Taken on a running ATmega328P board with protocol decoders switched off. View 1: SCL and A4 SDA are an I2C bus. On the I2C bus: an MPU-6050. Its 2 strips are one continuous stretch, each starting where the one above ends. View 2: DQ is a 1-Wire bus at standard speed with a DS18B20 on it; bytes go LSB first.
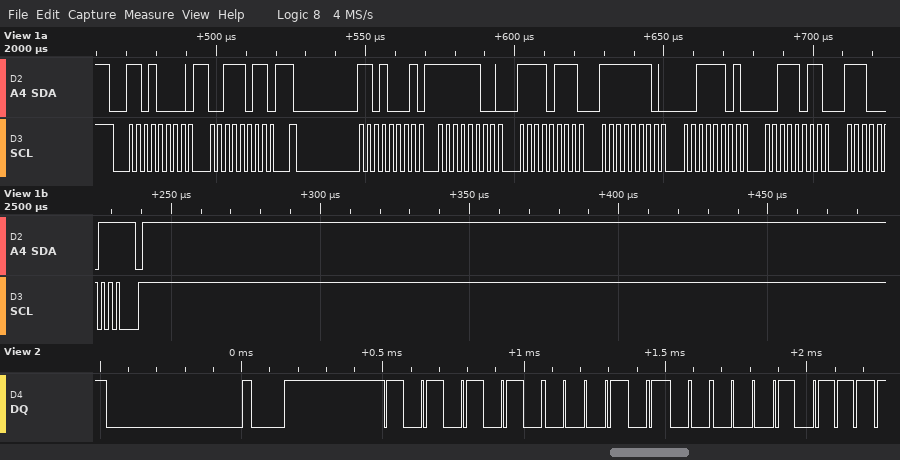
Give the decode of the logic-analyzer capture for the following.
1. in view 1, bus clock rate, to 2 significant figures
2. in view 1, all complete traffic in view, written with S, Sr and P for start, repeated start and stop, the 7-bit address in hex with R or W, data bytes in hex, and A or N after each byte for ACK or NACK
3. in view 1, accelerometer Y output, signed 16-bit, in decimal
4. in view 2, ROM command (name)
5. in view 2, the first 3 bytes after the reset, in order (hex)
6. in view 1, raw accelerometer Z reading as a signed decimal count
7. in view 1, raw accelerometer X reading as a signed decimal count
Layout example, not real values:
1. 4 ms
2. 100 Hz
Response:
1. 400 kHz
2. S 68W A 3B A Sr 68R A FC A F7 A FE A 3D A 3B A E3 N P
3. -451
4. Match ROM
5. 55 28 E8
6. 15331
7. -777
